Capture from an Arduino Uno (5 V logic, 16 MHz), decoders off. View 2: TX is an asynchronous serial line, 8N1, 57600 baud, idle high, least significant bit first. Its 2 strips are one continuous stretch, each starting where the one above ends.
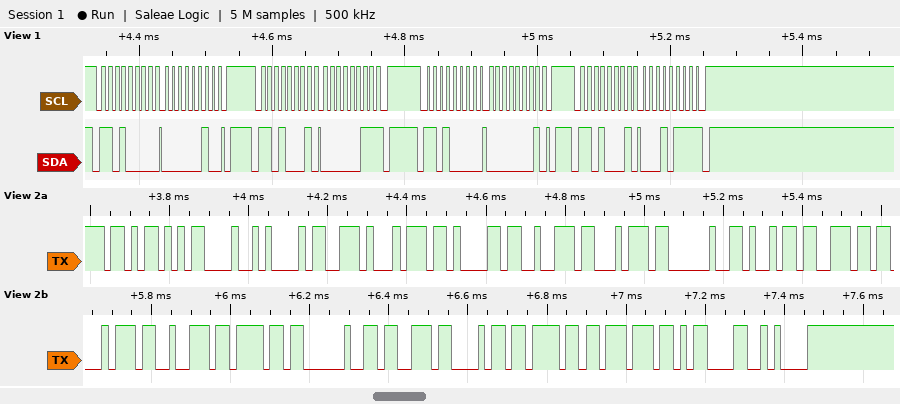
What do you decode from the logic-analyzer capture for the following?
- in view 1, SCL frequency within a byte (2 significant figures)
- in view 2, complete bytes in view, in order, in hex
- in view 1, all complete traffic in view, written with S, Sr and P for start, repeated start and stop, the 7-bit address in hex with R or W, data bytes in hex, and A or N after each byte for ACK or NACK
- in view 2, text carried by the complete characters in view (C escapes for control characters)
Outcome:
100 kHz
6B 0D 0A 73 74 61 72 74 20 69 6E 74 72 6F 20 73 68 6F 77 0D 0A
S 68W A 02 A P S 68R A 03 N P S 68W A 01 A P S 68R A 17 N P
"k\r\nstart intro show\r\n"
